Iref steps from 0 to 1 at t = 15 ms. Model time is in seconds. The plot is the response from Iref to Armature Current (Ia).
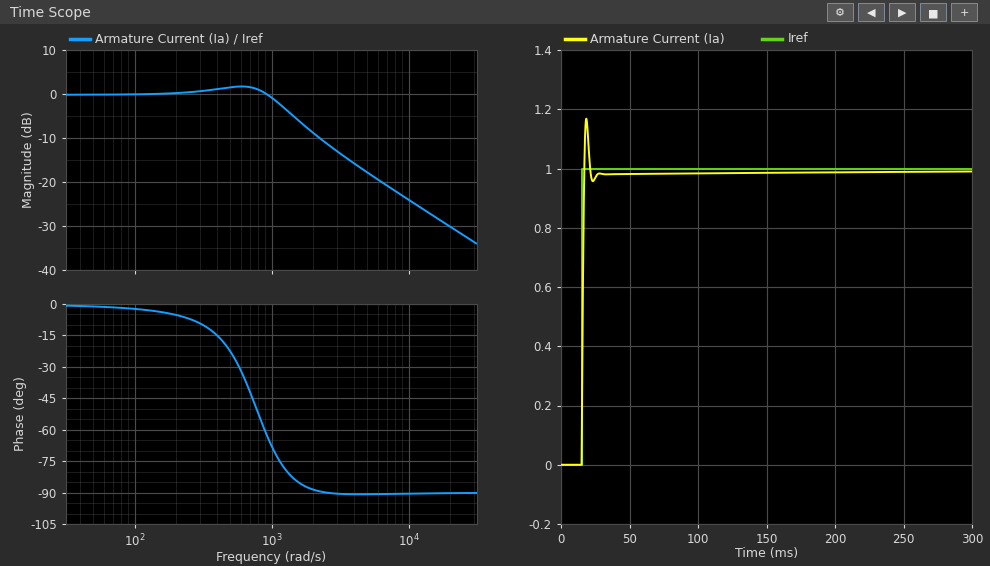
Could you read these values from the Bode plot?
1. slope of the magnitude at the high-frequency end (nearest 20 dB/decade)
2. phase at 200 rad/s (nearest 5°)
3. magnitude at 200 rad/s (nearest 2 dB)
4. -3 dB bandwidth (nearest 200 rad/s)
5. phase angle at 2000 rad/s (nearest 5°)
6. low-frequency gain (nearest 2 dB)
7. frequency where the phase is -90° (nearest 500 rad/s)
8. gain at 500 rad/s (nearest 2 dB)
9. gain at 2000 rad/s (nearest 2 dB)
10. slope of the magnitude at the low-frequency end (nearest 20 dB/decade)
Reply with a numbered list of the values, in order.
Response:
1. -20 dB/decade
2. -5°
3. 0 dB
4. 1200 rad/s
5. -90°
6. 0 dB
7. 2500 rad/s
8. 2 dB
9. -8 dB
10. 0 dB/decade
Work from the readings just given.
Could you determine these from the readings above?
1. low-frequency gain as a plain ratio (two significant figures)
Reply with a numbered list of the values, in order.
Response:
1. 1.0
